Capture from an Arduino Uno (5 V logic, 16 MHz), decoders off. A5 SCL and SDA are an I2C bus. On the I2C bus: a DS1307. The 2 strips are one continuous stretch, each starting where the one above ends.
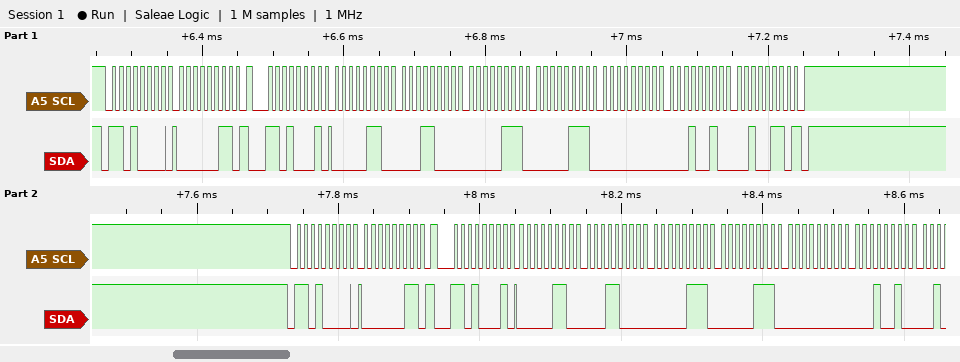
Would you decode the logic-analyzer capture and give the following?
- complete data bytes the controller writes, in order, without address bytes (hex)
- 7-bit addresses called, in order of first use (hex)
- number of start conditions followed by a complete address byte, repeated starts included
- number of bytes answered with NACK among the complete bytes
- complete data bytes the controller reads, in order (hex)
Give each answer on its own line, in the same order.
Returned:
03 03
0x68
4
1
06 18 07 07 00 12 26 06 18 07 07 00 12
